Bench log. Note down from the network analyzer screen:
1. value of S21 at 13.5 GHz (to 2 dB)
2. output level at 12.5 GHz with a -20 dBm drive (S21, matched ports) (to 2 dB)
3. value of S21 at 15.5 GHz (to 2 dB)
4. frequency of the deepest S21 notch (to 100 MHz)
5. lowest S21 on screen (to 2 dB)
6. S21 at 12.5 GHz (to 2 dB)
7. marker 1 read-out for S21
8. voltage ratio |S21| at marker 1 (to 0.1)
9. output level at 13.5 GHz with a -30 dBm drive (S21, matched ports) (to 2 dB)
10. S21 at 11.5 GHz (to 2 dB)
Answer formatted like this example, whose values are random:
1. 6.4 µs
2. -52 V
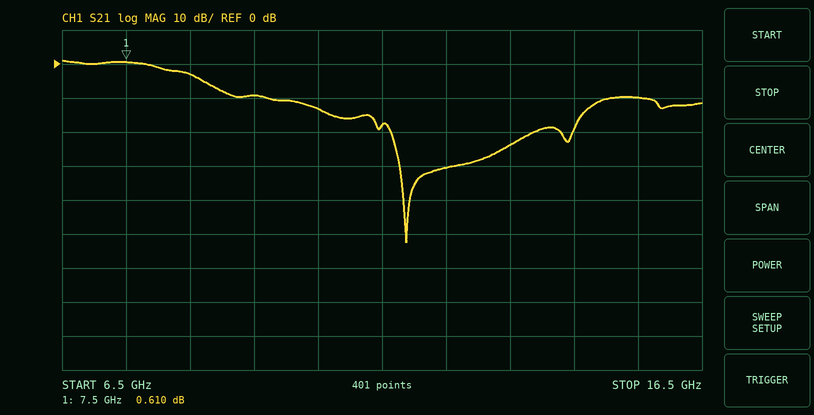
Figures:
1. -24 dB
2. -50 dBm
3. -10 dB
4. 11.9 GHz
5. -52 dB
6. -30 dB
7. 0.610 dB
8. 1.1
9. -54 dBm
10. -18 dB
